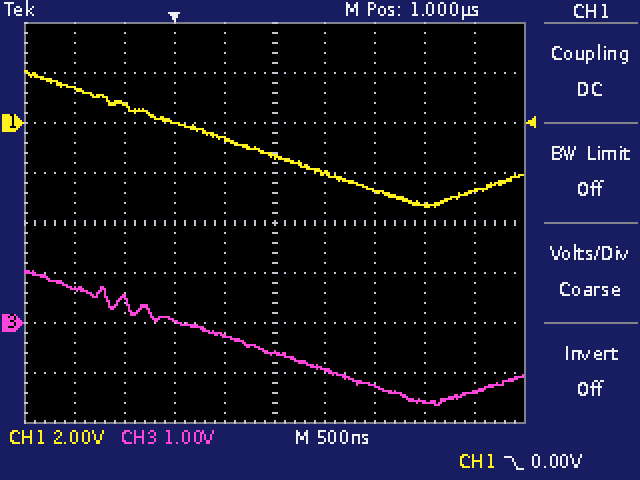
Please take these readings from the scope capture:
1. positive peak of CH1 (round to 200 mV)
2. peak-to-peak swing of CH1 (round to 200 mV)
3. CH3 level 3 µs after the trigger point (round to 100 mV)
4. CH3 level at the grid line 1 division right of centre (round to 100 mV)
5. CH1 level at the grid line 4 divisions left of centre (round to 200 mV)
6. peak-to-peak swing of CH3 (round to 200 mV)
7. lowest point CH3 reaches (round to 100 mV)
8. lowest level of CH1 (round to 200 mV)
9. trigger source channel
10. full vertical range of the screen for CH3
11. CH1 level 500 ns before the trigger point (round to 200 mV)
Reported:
2.0 V
5.4 V
-1.4 V
-900 mV
1.4 V
2.6 V
-1.6 V
-3.4 V
CH1
8 V
800 mV
